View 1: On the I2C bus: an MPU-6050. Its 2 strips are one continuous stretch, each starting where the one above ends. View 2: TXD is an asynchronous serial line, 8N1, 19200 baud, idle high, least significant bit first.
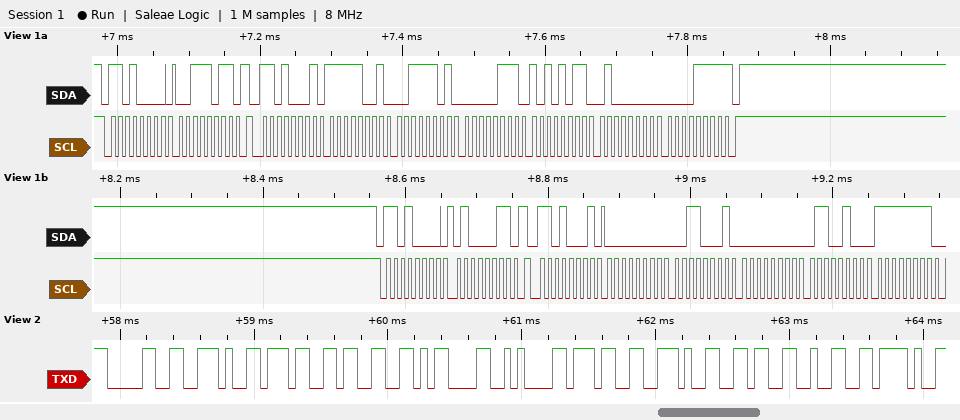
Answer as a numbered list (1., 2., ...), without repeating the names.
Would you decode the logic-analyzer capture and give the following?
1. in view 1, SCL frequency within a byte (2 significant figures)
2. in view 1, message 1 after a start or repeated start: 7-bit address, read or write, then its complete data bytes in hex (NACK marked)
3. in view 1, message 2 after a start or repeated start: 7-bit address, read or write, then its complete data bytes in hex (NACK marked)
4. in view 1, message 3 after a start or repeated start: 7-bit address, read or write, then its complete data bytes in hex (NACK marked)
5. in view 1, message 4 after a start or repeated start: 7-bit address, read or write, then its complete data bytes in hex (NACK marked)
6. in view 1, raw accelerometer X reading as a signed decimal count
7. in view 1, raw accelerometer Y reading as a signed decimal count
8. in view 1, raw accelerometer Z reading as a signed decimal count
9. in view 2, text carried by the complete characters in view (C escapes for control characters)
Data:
1. 100 kHz
2. 0x68 write: 3B
3. 0x68 read: F9 3D 07 AB 40 0F NACK
4. 0x68 write: 43
5. 0x68 read: 00 31 00 64 FF
6. -1731
7. 1963
8. 16399
9. "0.73\r\n7.62/"
